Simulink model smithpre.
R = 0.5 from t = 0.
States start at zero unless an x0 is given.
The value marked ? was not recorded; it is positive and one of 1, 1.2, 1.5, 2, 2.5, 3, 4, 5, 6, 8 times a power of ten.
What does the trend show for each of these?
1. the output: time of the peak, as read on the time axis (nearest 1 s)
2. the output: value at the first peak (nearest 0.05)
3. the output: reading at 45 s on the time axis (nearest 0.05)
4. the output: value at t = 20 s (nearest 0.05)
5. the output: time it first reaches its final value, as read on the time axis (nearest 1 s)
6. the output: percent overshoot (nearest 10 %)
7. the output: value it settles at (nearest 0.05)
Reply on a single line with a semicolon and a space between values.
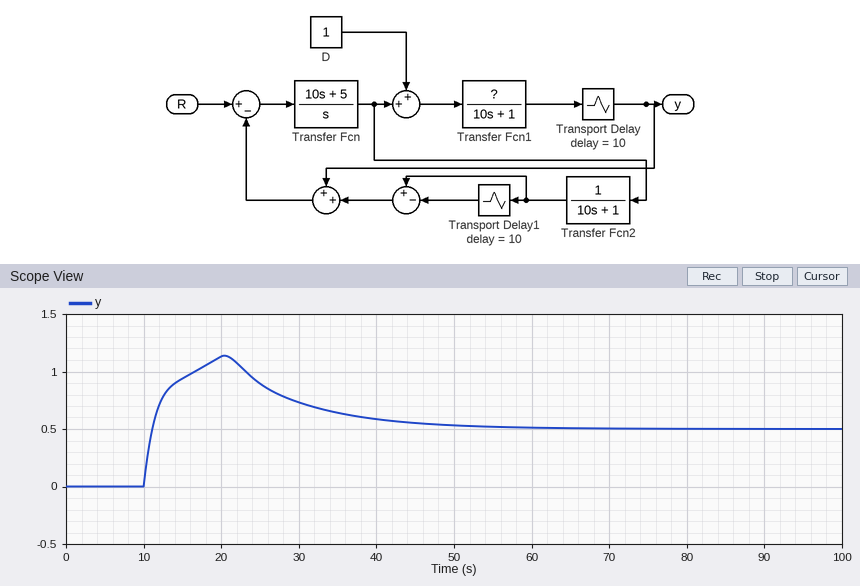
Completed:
20 s; 1.15; 0.55; 1.15; 11 s; 130 %; 0.50
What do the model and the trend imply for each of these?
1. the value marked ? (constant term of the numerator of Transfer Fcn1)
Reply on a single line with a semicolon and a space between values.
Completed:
1
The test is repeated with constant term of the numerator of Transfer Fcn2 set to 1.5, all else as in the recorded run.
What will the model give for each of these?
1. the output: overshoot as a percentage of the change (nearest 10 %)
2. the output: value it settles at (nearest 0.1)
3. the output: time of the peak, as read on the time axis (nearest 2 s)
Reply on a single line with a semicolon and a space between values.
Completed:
110 %; 0.5; 22 s
